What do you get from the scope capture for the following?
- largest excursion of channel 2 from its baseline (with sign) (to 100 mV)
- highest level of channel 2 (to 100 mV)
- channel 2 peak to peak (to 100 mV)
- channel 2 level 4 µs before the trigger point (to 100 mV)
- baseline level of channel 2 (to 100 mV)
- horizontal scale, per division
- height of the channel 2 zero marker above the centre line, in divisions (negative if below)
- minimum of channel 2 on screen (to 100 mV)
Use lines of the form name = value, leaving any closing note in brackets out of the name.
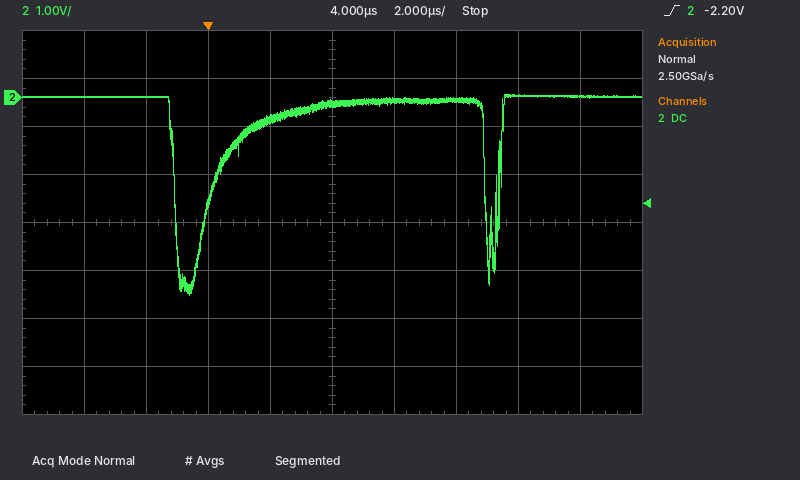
largest excursion of channel 2 from its baseline (with sign) = -4.1 V
highest level of channel 2 = 100 mV
channel 2 peak to peak = 4.2 V
channel 2 level 4 µs before the trigger point = 0.0 V
baseline level of channel 2 = 0.0 V
horizontal scale, per division = 2 µs
height of the channel 2 zero marker above the centre line, in divisions = +2.6 div
minimum of channel 2 on screen = -4.1 V
